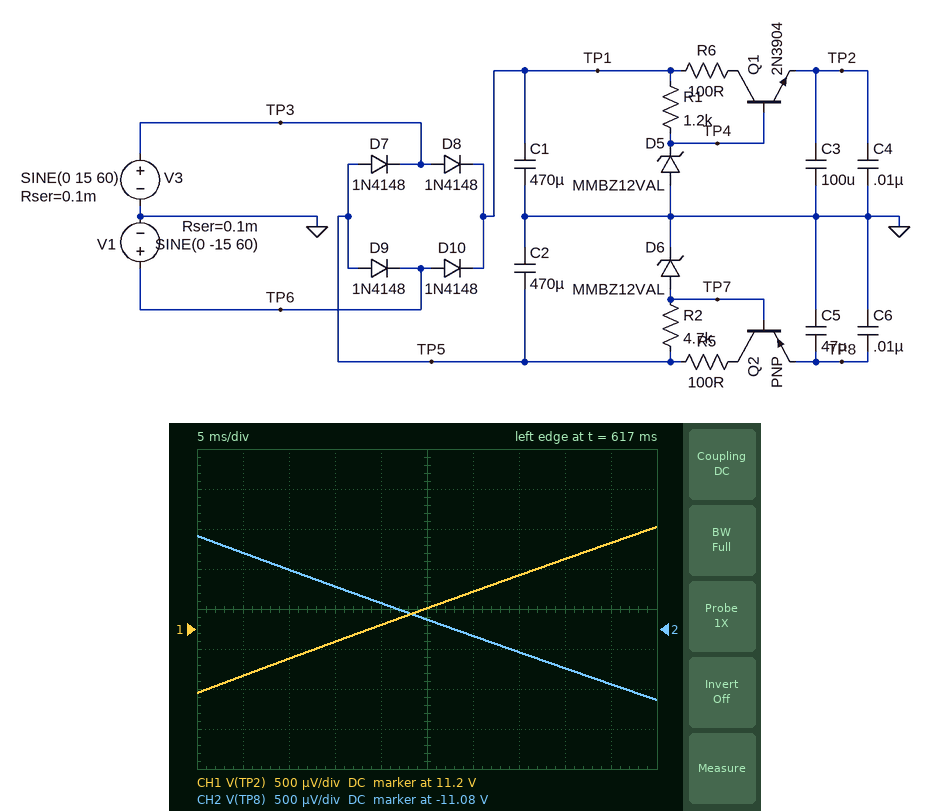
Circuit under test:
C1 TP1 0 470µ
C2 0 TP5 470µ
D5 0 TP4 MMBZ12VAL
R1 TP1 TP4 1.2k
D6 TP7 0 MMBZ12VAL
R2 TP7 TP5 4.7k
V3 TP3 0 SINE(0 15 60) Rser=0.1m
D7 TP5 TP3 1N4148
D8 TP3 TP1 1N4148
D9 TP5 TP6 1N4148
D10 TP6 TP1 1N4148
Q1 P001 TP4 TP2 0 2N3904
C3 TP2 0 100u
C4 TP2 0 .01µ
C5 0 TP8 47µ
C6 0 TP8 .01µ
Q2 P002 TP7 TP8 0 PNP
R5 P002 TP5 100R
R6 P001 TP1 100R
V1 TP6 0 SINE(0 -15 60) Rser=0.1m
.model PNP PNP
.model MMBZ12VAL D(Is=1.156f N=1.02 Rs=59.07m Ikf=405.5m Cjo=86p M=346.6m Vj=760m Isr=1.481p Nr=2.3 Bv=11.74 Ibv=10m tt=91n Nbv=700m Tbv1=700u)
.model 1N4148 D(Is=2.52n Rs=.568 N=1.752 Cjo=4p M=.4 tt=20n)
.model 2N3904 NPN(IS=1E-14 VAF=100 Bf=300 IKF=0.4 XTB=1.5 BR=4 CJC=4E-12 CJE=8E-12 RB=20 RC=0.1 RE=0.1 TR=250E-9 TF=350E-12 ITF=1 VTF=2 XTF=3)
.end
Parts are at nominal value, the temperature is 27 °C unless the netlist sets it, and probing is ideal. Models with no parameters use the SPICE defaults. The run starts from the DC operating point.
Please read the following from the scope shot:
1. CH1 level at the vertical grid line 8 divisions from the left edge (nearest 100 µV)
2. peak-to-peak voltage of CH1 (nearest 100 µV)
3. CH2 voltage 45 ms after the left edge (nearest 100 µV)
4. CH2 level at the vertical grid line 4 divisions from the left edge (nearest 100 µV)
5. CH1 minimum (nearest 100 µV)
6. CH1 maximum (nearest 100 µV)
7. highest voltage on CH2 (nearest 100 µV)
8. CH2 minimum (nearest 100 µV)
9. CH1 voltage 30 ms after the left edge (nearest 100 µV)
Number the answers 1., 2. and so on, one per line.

1. 11.1999 V
2. 2.1 mV
3. -11.0762 V
4. -11.0752 V
5. 11.1982 V
6. 11.2003 V
7. -11.0743 V
8. -11.0764 V
9. 11.1995 V
